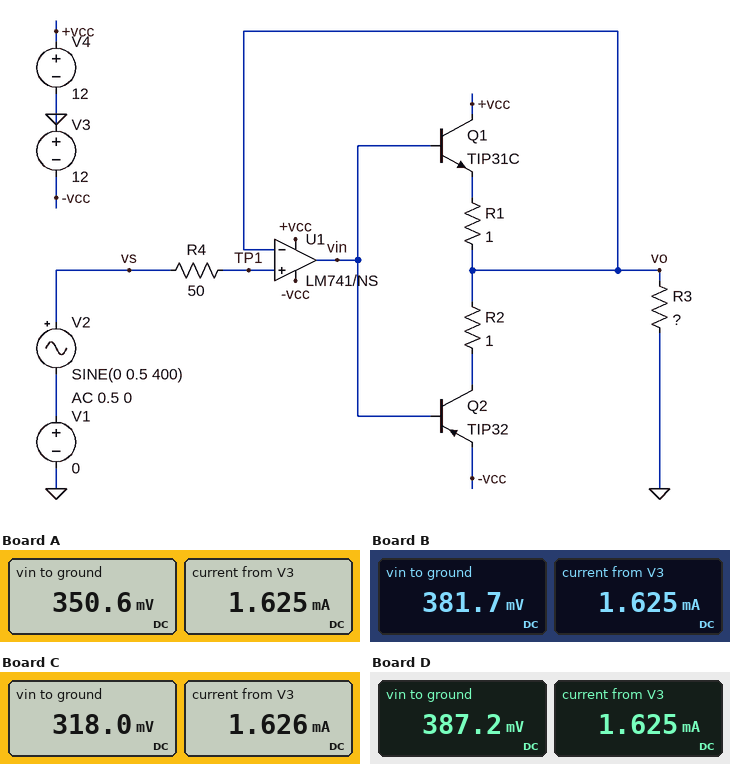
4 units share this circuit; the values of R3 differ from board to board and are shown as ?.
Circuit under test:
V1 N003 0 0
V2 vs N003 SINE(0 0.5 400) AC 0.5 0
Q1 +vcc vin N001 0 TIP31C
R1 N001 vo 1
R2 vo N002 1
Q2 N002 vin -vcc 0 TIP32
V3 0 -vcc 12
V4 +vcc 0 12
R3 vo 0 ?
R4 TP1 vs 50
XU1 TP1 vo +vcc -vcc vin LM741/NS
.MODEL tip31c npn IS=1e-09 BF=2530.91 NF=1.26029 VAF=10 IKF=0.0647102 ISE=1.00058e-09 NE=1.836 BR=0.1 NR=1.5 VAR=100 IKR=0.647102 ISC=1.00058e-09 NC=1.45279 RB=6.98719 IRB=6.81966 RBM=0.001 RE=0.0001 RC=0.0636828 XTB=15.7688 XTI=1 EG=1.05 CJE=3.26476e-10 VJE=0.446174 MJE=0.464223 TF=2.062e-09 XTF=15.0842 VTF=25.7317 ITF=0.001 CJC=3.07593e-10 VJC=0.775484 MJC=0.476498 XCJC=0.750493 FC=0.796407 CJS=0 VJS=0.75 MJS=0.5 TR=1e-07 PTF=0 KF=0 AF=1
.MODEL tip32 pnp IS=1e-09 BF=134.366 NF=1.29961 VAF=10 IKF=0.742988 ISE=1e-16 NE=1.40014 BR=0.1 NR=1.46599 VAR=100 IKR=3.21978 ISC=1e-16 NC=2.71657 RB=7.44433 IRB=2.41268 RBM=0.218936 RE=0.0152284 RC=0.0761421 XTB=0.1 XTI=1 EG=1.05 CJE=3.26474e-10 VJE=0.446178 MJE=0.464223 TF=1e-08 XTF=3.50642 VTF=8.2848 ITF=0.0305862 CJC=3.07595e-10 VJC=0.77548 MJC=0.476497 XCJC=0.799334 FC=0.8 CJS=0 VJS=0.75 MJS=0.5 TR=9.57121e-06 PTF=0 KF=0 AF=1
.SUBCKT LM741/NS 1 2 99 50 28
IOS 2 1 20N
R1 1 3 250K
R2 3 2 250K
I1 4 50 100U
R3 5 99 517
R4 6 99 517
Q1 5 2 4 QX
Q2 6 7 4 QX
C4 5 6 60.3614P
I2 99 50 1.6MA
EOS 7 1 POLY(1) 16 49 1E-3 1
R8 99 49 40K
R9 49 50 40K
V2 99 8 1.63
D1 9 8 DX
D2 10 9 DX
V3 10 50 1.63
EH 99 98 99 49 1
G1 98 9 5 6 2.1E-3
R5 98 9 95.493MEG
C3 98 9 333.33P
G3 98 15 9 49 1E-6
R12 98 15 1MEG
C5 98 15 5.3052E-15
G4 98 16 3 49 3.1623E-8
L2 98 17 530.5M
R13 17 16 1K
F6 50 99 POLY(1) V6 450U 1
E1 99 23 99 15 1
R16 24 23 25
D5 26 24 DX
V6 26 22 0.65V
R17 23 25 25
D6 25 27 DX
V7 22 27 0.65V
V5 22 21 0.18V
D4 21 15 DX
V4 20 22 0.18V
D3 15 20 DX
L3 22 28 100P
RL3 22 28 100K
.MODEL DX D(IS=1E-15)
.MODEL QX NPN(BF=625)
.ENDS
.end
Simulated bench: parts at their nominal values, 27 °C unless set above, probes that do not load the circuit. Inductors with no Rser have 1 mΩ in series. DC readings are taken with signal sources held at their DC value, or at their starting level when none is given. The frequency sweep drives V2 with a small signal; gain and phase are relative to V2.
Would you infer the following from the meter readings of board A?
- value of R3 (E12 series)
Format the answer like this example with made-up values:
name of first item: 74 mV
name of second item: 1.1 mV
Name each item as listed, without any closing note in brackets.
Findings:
value of R3: 10 Ω
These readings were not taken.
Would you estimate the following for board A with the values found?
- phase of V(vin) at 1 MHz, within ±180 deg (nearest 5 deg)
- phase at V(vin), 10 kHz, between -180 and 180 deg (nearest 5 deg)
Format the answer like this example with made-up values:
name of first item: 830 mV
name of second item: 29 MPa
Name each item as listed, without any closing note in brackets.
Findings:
phase of V(vin) at 1 MHz, within ±180 deg: -155 deg
phase at V(vin), 10 kHz, between -180 and 180 deg: -20 deg
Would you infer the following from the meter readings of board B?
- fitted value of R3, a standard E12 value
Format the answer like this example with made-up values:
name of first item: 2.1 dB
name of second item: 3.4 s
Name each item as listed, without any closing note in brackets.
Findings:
fitted value of R3, a standard E12 value: 3.9 Ω
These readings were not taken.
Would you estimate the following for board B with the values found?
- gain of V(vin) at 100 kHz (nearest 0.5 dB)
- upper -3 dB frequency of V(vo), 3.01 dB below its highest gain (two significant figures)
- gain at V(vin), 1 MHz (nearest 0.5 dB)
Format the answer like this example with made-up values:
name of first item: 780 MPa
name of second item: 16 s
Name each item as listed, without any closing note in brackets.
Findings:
gain of V(vin) at 100 kHz: 19.5 dB
upper -3 dB frequency of V(vo), 3.01 dB below its highest gain: 30 kHz
gain at V(vin), 1 MHz: -5.0 dB
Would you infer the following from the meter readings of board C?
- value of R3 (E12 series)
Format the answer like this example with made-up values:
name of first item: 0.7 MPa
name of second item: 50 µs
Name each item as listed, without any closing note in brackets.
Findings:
value of R3: 27 Ω
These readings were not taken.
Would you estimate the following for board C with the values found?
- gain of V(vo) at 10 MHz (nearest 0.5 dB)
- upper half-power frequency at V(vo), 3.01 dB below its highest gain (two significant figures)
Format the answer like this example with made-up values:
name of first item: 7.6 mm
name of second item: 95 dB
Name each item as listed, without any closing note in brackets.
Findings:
gain of V(vo) at 10 MHz: -51.0 dB
upper half-power frequency at V(vo), 3.01 dB below its highest gain: 27 kHz
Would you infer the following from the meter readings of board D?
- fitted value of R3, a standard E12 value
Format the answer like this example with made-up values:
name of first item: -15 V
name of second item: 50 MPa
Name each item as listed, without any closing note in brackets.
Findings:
fitted value of R3, a standard E12 value: 3.3 Ω
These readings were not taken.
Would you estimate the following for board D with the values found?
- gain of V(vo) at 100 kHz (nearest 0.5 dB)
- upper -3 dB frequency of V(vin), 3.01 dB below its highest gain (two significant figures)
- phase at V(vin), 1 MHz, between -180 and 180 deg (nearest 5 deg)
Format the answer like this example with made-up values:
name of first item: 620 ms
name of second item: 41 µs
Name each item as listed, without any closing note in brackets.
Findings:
gain of V(vo) at 100 kHz: -11.0 dB
upper -3 dB frequency of V(vin), 3.01 dB below its highest gain: 30 kHz
phase at V(vin), 1 MHz, between -180 and 180 deg: -160 deg
